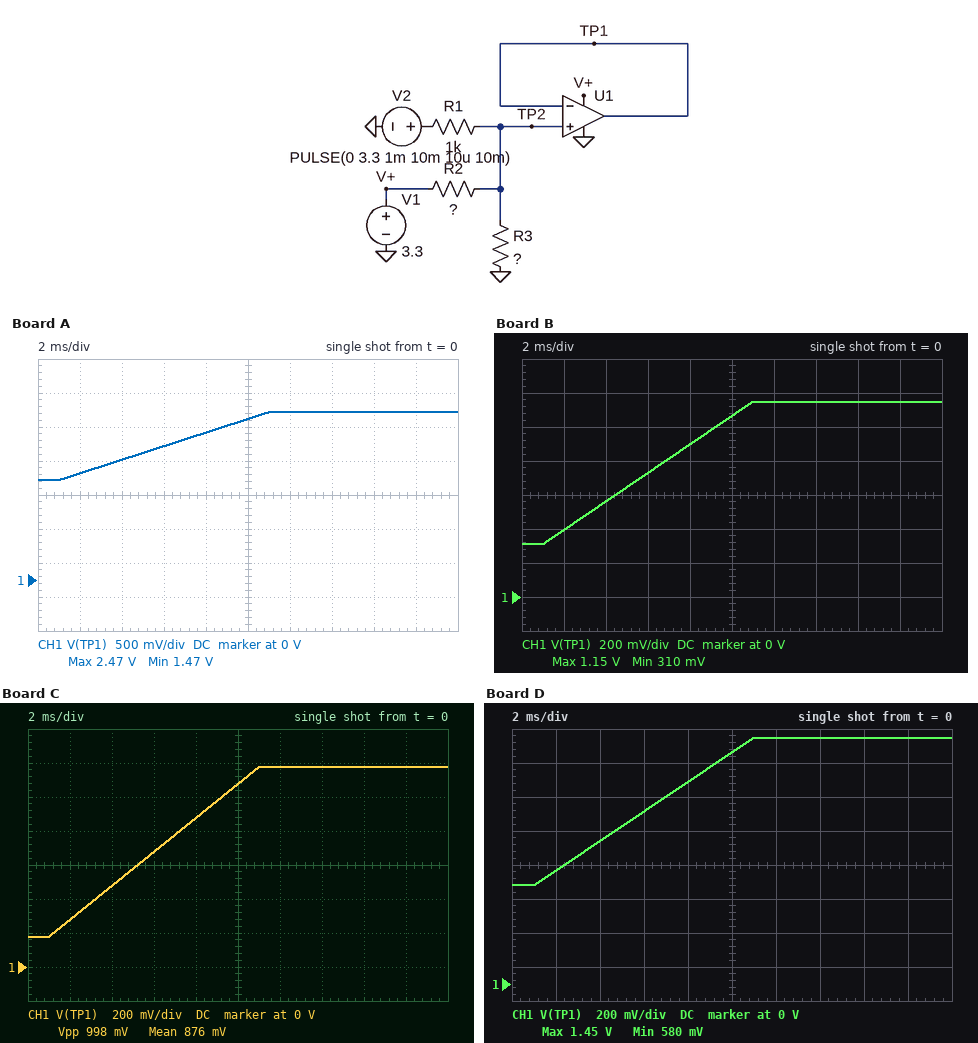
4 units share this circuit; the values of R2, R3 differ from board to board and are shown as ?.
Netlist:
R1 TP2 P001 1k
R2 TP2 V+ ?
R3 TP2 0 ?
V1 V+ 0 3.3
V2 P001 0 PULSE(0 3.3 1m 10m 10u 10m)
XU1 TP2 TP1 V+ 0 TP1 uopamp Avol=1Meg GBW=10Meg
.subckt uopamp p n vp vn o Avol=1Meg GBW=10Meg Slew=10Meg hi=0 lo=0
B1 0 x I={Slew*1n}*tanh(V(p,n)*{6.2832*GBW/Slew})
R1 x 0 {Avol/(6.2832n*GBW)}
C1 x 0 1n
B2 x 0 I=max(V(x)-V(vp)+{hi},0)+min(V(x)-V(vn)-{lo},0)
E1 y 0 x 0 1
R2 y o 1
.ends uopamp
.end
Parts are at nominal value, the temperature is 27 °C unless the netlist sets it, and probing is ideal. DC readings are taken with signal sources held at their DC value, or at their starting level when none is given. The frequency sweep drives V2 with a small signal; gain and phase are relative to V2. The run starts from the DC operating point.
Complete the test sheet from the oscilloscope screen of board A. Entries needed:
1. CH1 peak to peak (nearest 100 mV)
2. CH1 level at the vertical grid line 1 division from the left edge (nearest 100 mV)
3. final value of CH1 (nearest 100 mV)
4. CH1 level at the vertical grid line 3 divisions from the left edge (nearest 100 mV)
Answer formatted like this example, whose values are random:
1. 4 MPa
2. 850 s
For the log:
1. 1.0 V
2. 1.6 V
3. 2.5 V
4. 2.0 V
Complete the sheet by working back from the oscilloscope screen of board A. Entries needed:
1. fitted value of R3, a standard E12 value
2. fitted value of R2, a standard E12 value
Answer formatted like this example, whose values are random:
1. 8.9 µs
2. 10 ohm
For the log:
1. 1.2 kΩ
2. 680 Ω
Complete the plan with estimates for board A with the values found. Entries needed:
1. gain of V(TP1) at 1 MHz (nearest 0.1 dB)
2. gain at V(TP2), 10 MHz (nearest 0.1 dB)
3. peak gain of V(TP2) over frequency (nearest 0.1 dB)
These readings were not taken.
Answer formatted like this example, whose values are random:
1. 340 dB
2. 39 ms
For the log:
1. -10.4 dB
2. -10.4 dB
3. -10.4 dB
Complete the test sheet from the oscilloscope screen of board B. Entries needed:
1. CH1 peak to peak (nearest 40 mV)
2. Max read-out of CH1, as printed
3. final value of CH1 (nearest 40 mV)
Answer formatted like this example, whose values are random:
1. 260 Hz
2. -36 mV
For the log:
1. 840 mV
2. 1.15 V
3. 1.16 V
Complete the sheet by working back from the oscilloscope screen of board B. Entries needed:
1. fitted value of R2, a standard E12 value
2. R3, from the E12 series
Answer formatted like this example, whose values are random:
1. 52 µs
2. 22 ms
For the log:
1. 2.7 kΩ
2. 390 Ω
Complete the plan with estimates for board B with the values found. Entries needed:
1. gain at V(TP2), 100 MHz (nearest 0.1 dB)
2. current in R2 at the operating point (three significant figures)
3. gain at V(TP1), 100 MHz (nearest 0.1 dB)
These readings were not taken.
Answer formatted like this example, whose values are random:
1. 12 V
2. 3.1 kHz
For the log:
1. -11.9 dB
2. 1.11 mA
3. -31.9 dB
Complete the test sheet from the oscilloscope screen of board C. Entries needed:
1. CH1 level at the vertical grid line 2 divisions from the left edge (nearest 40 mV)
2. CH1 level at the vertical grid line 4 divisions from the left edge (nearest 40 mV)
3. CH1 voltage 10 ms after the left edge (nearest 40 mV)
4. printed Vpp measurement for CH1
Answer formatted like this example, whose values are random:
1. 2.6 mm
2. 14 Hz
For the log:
1. 480 mV
2. 880 mV
3. 1.08 V
4. 998 mV
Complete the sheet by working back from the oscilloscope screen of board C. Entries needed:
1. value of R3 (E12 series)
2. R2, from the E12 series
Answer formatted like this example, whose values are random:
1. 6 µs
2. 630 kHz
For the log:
1. 470 Ω
2. 5.6 kΩ
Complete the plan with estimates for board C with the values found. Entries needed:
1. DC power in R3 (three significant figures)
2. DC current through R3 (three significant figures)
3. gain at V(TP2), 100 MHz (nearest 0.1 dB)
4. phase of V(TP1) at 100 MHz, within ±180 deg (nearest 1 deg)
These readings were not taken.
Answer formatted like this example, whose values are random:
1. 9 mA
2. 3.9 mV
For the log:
1. 67.6 µW
2. 379 µA
3. -10.4 dB
4. -84 deg
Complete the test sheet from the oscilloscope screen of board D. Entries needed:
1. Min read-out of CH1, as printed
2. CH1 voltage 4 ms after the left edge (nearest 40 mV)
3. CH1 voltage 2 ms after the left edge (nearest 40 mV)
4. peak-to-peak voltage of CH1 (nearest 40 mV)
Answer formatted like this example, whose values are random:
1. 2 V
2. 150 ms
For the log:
1. 580 mV
2. 840 mV
3. 680 mV
4. 880 mV
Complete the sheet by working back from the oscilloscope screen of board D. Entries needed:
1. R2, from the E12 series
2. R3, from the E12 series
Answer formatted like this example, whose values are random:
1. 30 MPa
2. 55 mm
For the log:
1. 1.5 kΩ
2. 470 Ω
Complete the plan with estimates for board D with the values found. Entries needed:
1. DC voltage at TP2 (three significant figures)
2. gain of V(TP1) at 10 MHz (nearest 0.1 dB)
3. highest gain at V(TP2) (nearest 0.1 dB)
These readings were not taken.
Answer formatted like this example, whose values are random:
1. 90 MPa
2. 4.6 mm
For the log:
1. 580 mV
2. -14.6 dB
3. -11.6 dB
